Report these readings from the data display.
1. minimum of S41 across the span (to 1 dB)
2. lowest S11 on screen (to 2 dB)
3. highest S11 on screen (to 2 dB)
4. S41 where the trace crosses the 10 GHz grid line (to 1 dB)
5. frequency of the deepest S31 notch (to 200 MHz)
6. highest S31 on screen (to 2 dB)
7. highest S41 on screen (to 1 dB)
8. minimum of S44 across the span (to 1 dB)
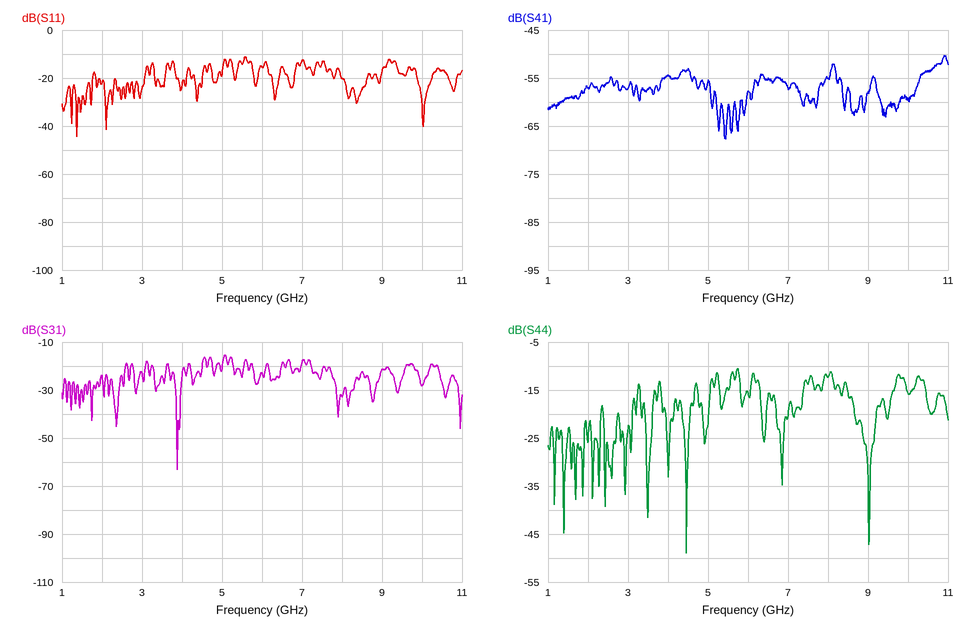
-68 dB
-44 dB
-12 dB
-59 dB
3.8 GHz
-16 dB
-50 dB
-49 dB
